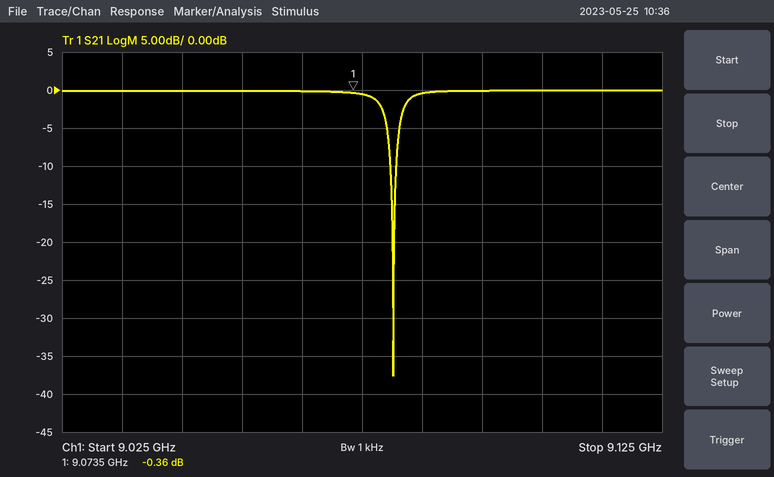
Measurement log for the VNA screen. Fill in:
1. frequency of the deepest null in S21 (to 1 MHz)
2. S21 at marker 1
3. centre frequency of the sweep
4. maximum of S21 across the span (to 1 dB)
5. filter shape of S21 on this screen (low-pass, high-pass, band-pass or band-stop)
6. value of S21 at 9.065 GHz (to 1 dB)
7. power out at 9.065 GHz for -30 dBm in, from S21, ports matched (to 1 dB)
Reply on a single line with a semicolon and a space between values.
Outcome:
9.080 GHz; -0.36 dB; 9.075 GHz; 0 dB; band-stop; 0 dB; -30 dBm
